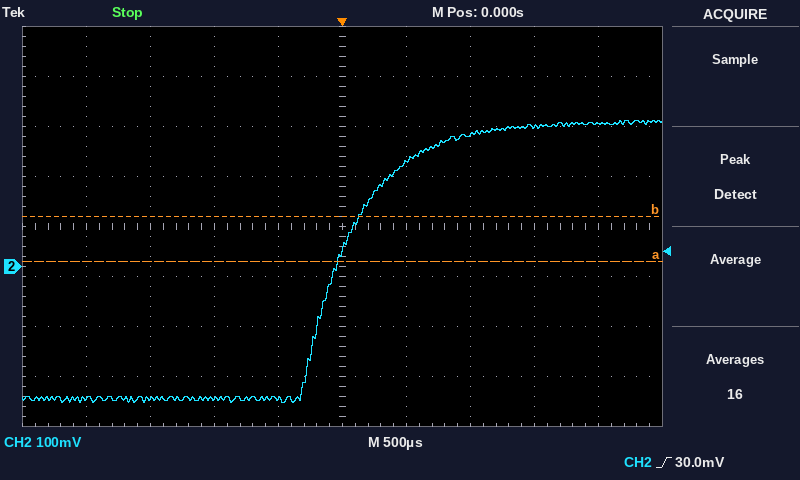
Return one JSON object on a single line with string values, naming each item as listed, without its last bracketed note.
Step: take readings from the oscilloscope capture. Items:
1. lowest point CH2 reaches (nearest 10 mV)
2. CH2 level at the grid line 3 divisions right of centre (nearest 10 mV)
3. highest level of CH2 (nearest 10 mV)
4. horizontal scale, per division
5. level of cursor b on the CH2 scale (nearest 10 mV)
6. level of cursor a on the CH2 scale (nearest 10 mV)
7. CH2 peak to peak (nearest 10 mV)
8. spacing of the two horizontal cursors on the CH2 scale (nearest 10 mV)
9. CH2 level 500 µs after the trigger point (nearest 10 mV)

{"lowest point CH2 reaches": "-270 mV", "CH2 level at the grid line 3 divisions right of centre": "280 mV", "highest level of CH2": "290 mV", "horizontal scale, per division": "500 µs", "level of cursor b on the CH2 scale": "100 mV", "level of cursor a on the CH2 scale": "10 mV", "CH2 peak to peak": "560 mV", "spacing of the two horizontal cursors on the CH2 scale": "90 mV", "CH2 level 500 µs after the trigger point": "210 mV"}
